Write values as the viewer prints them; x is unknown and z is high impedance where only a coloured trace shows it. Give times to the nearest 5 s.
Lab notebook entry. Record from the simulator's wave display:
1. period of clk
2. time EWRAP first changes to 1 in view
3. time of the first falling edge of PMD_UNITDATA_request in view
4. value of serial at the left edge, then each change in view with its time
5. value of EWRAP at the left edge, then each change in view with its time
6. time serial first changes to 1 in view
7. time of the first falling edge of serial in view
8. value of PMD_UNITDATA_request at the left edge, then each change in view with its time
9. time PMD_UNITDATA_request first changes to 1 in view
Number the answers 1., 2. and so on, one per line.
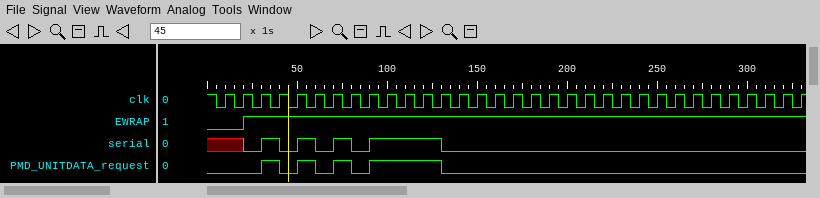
1. 10 s
2. 20 s
3. 40 s
4. x, 0 at 20 s, 1 at 30 s, 0 at 40 s, 1 at 50 s, 0 at 60 s, 1 at 70 s, 0 at 80 s, 1 at 90 s, 0 at 130 s
5. 0, 1 at 20 s
6. 30 s
7. 40 s
8. 0, 1 at 30 s, 0 at 40 s, 1 at 50 s, 0 at 60 s, 1 at 70 s, 0 at 80 s, 1 at 90 s, 0 at 130 s
9. 30 s
